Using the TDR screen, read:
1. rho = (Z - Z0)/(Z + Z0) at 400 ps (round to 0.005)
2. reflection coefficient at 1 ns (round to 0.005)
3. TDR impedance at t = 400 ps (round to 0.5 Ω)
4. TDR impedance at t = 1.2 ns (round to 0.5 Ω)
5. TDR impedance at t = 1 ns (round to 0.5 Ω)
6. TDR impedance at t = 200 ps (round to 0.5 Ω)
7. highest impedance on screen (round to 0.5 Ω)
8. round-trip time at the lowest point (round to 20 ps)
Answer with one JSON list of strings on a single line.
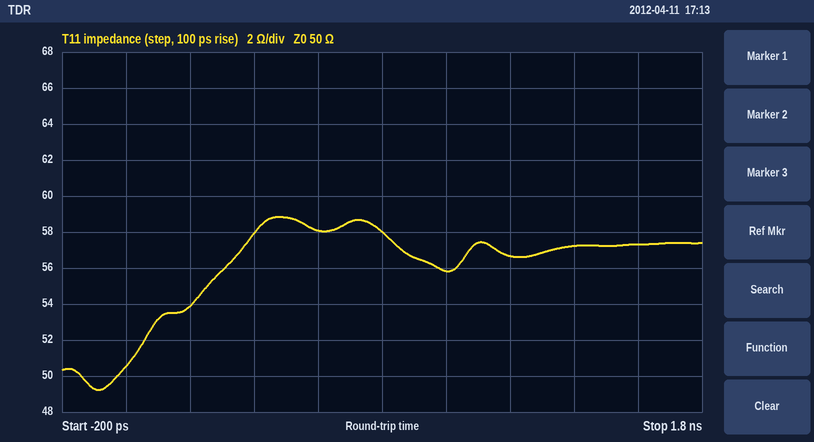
["+0.075", "+0.055", "58.0 Ω", "56.5 Ω", "56.0 Ω", "54.0 Ω", "59.0 Ω", "-80 ps"]
